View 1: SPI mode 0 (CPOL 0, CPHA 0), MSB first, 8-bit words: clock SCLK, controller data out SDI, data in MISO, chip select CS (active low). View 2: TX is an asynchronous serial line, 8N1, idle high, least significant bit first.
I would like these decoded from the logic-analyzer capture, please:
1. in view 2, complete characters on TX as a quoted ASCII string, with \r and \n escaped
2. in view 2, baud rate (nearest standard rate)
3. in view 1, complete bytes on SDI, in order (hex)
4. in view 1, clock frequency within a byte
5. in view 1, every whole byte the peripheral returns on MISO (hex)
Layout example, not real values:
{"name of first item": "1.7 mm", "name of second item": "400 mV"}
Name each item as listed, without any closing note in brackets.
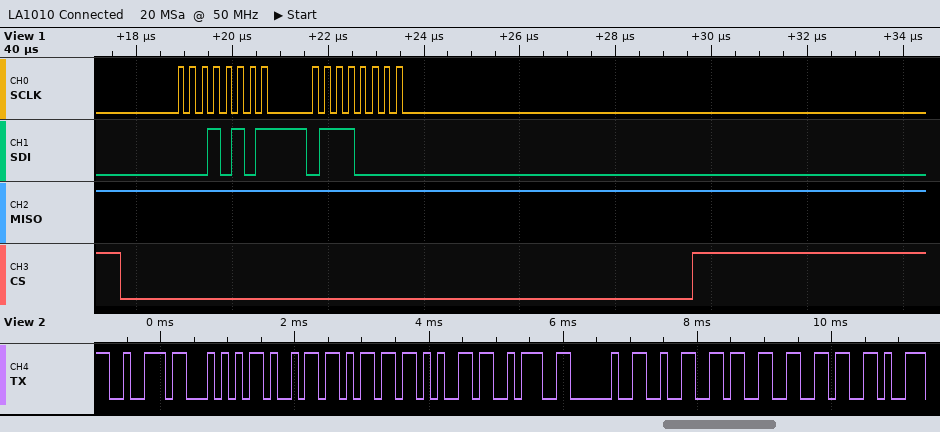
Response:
{"in view 2, complete characters on TX as a quoted ASCII string, with \\r and \\n escaped": "\"rTime: 236\"", "in view 2, baud rate": "9600 baud", "in view 1, complete bytes on SDI, in order": "15 70", "in view 1, clock frequency within a byte": "4 MHz", "in view 1, every whole byte the peripheral returns on MISO": "FF FF"}
